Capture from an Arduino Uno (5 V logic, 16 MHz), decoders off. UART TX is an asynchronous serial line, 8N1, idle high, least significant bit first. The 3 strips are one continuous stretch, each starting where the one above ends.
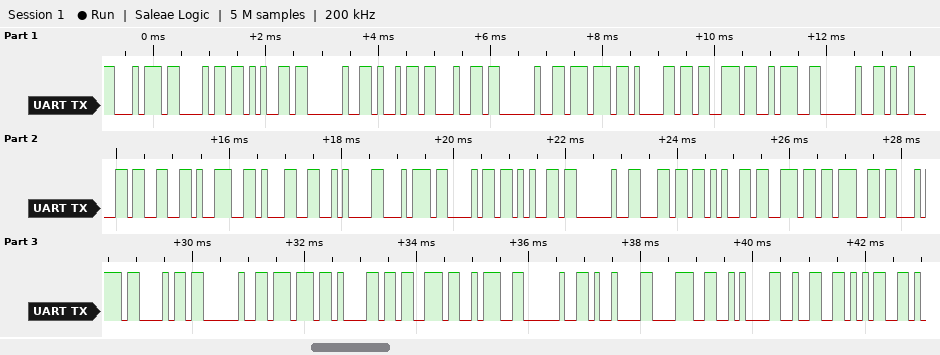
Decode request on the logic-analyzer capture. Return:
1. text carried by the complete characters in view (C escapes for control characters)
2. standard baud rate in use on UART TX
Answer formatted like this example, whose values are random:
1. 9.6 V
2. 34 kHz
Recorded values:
1. "the id was: \t391\nthe length was: \t8\n25"
2. 9600 baud
